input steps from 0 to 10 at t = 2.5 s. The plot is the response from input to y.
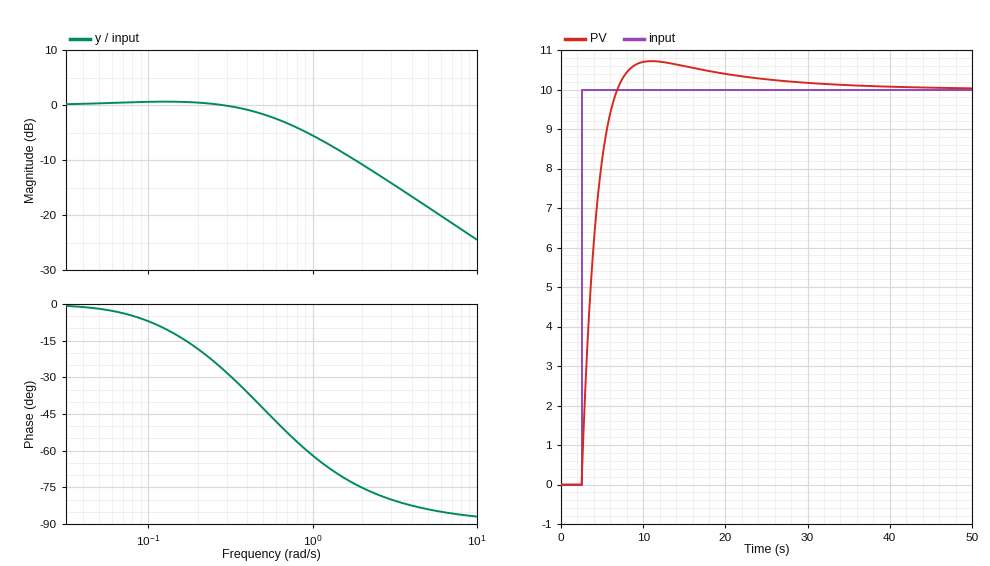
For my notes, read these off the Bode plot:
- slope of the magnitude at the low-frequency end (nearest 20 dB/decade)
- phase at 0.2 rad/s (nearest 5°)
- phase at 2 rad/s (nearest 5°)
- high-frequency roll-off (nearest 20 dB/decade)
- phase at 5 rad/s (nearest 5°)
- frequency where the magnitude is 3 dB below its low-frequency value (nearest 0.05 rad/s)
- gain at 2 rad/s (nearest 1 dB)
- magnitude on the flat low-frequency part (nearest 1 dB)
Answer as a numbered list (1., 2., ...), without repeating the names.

1. 0 dB/decade
2. -20°
3. -75°
4. -20 dB/decade
5. -85°
6. 0.65 rad/s
7. -11 dB
8. 0 dB
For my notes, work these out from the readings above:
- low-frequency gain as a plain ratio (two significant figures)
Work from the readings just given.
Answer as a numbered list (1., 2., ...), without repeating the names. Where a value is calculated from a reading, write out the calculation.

1. 10^(0 / 20) = 1.0
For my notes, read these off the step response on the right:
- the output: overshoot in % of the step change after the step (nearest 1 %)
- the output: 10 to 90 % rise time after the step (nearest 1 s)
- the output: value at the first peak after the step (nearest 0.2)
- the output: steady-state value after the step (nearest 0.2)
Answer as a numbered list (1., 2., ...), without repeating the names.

1. 7 %
2. 3 s
3. 10.8
4. 10.0
